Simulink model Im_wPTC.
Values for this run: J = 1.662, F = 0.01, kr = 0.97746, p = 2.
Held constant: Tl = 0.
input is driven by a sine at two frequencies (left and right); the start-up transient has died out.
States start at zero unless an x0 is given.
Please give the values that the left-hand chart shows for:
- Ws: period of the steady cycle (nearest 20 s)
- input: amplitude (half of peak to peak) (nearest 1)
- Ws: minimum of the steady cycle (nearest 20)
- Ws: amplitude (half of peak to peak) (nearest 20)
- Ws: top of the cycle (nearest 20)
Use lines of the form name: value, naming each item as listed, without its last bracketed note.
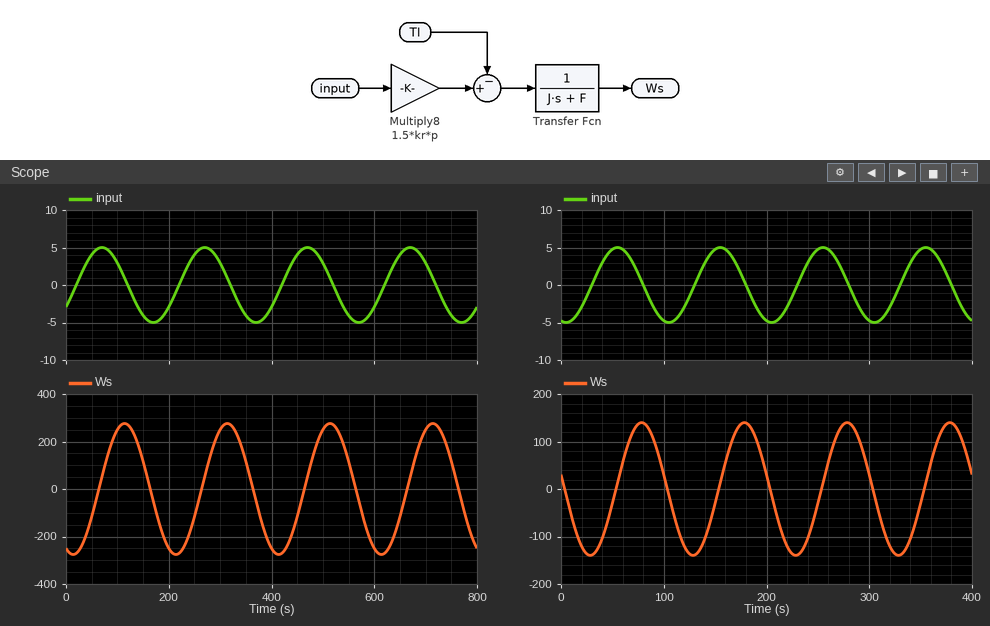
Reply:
Ws: period of the steady cycle: 200 s
input: amplitude (half of peak to peak): 5
Ws: minimum of the steady cycle: -280
Ws: amplitude (half of peak to peak): 280
Ws: top of the cycle: 280
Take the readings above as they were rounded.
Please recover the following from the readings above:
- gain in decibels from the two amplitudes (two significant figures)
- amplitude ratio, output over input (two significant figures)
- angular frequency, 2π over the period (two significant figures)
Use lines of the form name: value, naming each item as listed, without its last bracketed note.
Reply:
gain in decibels from the two amplitudes: 35 dB
amplitude ratio, output over input: 56
angular frequency, 2π over the period: 0.031 rad/s
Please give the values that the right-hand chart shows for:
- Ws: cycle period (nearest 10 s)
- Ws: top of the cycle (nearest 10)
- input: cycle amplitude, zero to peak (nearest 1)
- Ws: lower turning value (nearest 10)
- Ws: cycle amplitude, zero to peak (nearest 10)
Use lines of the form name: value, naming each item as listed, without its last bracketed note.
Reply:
Ws: cycle period: 100 s
Ws: top of the cycle: 140
input: cycle amplitude, zero to peak: 5
Ws: lower turning value: -140
Ws: cycle amplitude, zero to peak: 140
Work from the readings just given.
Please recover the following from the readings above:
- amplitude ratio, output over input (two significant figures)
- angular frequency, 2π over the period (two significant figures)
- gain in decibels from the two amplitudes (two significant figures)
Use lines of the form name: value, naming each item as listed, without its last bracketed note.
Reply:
amplitude ratio, output over input: 28
angular frequency, 2π over the period: 0.063 rad/s
gain in decibels from the two amplitudes: 29 dB
